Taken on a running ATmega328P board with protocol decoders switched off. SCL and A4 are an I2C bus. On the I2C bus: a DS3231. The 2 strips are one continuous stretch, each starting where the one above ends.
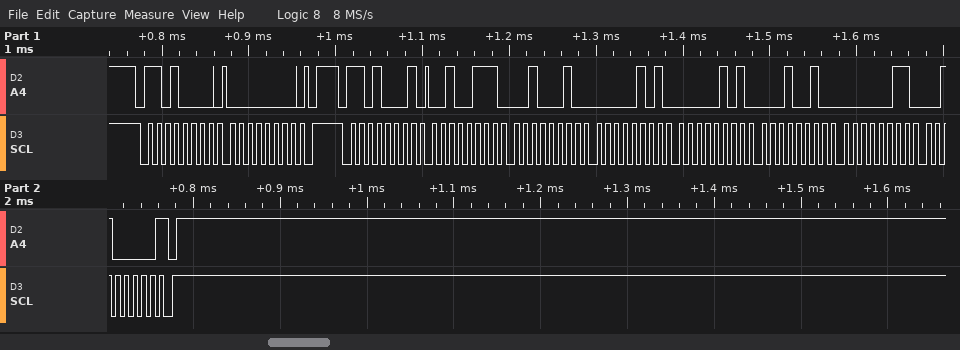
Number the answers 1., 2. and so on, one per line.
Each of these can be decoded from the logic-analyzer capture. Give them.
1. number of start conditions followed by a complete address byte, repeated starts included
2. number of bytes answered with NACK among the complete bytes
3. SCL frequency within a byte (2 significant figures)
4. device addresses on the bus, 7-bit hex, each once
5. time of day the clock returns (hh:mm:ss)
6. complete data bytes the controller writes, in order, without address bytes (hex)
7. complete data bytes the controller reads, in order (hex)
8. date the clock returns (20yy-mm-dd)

1. 2
2. 1
3. 100 kHz
4. 0x68
5. 05:22:27
6. 00
7. 27 22 05 05 12 03 20
8. 2020-03-12
